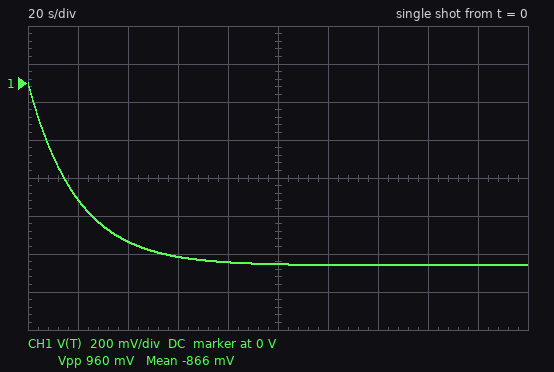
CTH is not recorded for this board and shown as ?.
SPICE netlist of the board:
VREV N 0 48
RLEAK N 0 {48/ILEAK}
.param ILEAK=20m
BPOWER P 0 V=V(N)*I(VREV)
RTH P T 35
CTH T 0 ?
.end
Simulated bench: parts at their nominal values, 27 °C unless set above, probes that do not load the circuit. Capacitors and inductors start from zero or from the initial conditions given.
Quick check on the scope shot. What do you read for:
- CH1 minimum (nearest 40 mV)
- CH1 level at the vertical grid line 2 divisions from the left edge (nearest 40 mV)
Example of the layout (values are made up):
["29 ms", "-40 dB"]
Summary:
["-960 mV", "-840 mV"]
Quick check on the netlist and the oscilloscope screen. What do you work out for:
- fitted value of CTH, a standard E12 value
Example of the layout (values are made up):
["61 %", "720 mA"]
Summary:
["560 mF"]
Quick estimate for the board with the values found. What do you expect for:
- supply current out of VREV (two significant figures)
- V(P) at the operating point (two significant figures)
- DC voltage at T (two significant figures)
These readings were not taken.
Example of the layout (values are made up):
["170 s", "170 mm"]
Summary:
["20 mA", "-960 mV", "-960 mV"]
